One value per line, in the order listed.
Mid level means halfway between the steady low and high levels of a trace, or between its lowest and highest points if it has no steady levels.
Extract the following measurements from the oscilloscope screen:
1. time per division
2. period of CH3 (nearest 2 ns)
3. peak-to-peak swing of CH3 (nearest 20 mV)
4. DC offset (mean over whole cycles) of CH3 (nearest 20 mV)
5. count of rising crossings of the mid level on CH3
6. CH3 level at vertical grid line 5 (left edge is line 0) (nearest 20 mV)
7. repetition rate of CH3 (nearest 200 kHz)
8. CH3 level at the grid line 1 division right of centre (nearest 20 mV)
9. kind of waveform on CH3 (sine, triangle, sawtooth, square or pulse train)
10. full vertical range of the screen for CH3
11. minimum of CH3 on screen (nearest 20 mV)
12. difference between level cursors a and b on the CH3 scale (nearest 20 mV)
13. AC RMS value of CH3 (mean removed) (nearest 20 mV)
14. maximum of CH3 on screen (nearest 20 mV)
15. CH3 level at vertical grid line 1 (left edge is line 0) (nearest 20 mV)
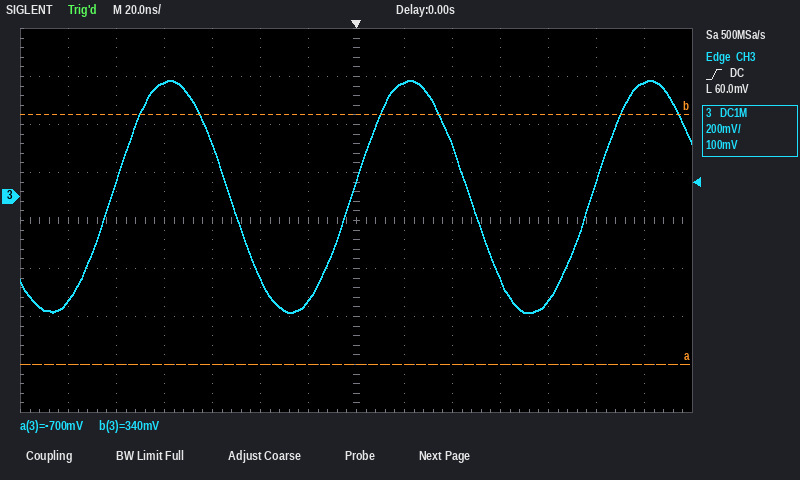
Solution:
20 ns
100 ns
960 mV
0 mV
3
-340 mV
10.0 MHz
480 mV
sine
1.6 V
-480 mV
1.04 V
340 mV
480 mV
-440 mV
